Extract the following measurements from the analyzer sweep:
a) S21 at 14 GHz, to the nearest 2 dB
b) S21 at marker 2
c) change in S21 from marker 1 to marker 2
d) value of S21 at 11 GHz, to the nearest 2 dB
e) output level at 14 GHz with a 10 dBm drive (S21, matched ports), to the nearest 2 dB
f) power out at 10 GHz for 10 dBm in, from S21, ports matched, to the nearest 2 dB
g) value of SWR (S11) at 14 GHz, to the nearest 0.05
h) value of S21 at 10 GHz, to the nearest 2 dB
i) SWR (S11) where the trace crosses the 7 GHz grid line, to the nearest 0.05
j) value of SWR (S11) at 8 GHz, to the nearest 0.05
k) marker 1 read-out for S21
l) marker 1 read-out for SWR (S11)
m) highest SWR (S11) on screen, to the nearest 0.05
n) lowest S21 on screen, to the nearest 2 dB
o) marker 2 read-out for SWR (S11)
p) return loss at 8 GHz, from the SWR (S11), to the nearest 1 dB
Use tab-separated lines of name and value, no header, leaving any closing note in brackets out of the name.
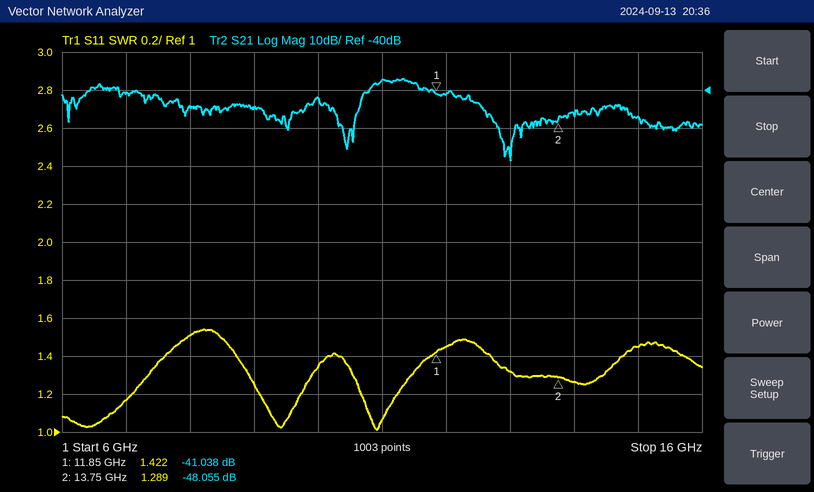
S21 at 14 GHz, to the nearest 2 dB	-46 dB
S21 at marker 2	-48.055 dB
change in S21 from marker 1 to marker 2	-7.017 dB
value of S21 at 11 GHz, to the nearest 2 dB	-38 dB
output level at 14 GHz with a 10 dBm drive (S21, matched ports), to the nearest 2 dB	-36 dBm
power out at 10 GHz for 10 dBm in, from S21, ports matched, to the nearest 2 dB	-32 dBm
value of SWR (S11) at 14 GHz, to the nearest 0.05	1.25
value of S21 at 10 GHz, to the nearest 2 dB	-42 dB
SWR (S11) where the trace crosses the 7 GHz grid line, to the nearest 0.05	1.15
value of SWR (S11) at 8 GHz, to the nearest 0.05	1.50
marker 1 read-out for S21	-41.038 dB
marker 1 read-out for SWR	1.422
highest SWR (S11) on screen, to the nearest 0.05	1.55
lowest S21 on screen, to the nearest 2 dB	-58 dB
marker 2 read-out for SWR	1.289
return loss at 8 GHz, from the SWR (S11), to the nearest 1 dB	14 dB
